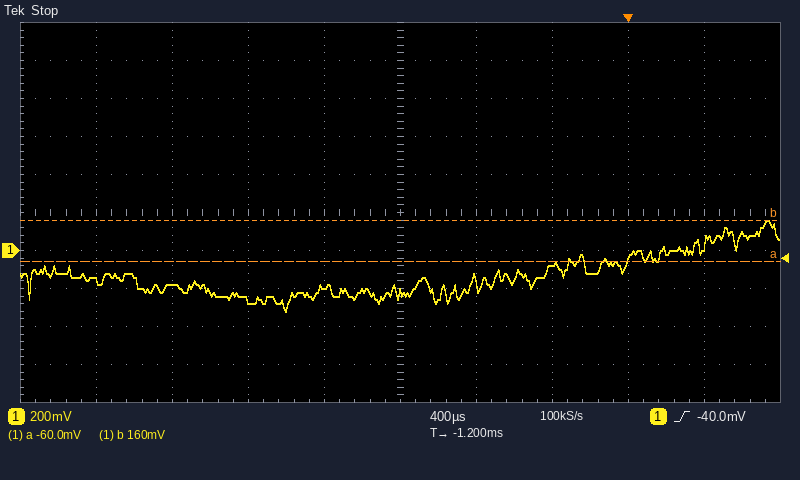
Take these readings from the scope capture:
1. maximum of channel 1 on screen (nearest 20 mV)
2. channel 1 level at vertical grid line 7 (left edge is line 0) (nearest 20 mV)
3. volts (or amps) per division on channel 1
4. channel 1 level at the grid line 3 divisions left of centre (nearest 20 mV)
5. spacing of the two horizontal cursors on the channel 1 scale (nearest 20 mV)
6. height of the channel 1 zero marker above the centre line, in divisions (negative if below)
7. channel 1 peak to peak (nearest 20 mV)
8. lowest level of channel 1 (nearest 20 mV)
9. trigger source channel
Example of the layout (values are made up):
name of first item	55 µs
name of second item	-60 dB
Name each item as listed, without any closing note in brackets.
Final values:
maximum of channel 1 on screen	160 mV
channel 1 level at vertical grid line 7 (left edge is line 0)	-80 mV
volts (or amps) per division on channel 1	200 mV
channel 1 level at the grid line 3 divisions left of centre	-180 mV
spacing of the two horizontal cursors on the channel 1 scale	220 mV
height of the channel 1 zero marker above the centre line, in divisions	-1.0 div
channel 1 peak to peak	480 mV
lowest level of channel 1	-320 mV
trigger source channel	channel 1
